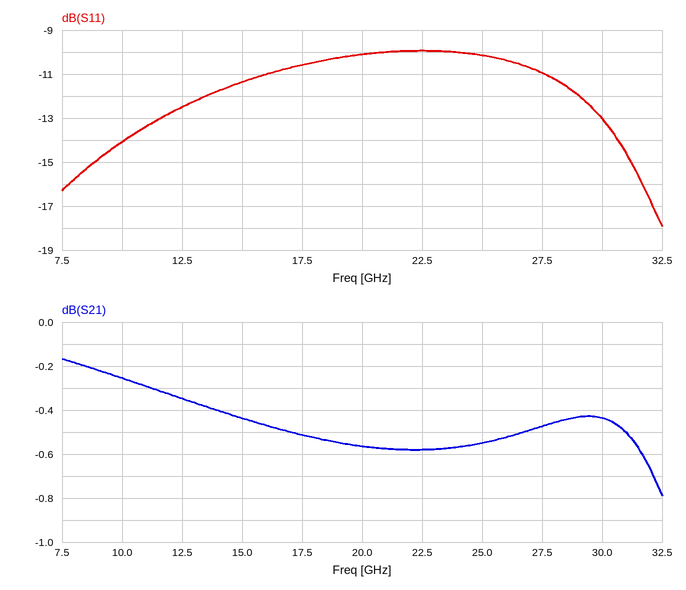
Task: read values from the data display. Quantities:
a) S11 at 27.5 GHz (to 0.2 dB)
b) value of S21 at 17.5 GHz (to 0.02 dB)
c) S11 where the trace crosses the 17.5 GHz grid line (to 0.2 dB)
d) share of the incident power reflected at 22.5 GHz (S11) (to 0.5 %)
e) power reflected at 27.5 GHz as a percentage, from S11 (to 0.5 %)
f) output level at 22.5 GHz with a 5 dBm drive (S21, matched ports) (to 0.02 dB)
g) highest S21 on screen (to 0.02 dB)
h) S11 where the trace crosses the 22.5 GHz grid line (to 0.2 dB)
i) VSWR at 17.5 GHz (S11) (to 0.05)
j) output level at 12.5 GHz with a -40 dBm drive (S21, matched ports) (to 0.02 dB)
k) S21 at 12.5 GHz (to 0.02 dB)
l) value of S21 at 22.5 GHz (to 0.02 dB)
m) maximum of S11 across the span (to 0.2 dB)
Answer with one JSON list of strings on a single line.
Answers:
["-11.0 dB", "-0.52 dB", "-10.6 dB", "10.0 %", "8.0 %", "4.42 dBm", "-0.16 dB", "-10.0 dB", "1.85", "-40.34 dBm", "-0.34 dB", "-0.58 dB", "-10.0 dB"]
